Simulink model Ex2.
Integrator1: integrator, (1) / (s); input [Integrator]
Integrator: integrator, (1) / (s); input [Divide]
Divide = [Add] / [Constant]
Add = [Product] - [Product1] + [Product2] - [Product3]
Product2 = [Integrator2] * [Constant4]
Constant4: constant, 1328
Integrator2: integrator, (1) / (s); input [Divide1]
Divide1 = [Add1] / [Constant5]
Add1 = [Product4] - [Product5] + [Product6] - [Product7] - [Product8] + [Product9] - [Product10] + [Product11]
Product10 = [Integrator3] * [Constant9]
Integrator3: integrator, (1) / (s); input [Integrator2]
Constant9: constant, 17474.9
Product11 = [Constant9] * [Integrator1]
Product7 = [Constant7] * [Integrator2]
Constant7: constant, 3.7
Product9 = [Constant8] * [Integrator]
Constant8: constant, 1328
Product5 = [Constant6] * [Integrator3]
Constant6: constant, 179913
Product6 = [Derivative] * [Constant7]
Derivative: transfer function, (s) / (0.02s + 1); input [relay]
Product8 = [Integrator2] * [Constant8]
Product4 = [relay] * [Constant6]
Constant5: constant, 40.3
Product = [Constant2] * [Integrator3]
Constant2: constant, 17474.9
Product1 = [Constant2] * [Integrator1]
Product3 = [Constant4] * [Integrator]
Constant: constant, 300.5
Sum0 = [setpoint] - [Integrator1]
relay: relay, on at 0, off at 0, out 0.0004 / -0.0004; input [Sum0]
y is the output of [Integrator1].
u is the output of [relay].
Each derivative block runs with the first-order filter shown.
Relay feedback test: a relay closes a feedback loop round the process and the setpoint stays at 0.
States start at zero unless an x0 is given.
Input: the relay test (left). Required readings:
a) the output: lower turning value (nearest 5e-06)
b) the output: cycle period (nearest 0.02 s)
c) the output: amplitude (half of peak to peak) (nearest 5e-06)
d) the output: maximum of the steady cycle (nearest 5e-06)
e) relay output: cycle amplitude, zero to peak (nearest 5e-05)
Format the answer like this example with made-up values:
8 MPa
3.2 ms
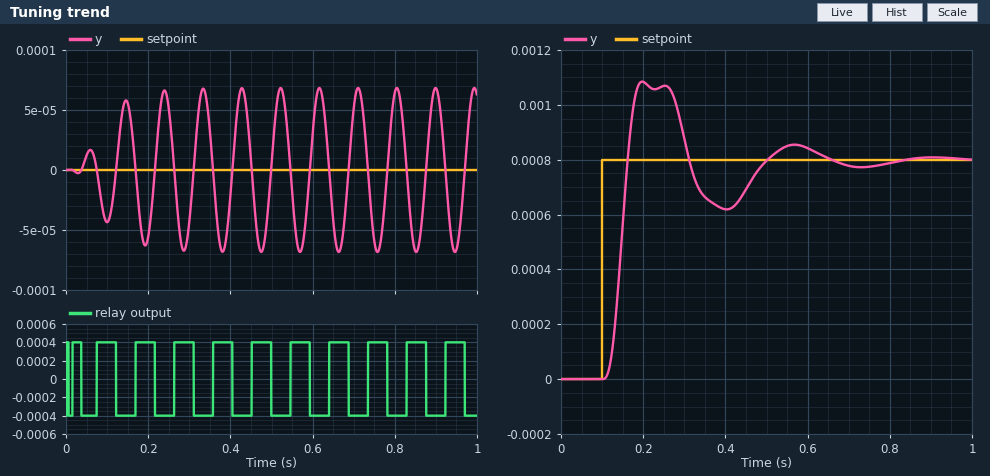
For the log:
-0.000070
0.10 s
0.000070
0.000070
0.00040
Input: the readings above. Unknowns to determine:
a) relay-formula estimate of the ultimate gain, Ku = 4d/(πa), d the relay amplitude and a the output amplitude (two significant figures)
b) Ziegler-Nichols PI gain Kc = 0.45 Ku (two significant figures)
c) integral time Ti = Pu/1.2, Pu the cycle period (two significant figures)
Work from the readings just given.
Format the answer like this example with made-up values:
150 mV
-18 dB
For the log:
7.3
3.3
0.083 s
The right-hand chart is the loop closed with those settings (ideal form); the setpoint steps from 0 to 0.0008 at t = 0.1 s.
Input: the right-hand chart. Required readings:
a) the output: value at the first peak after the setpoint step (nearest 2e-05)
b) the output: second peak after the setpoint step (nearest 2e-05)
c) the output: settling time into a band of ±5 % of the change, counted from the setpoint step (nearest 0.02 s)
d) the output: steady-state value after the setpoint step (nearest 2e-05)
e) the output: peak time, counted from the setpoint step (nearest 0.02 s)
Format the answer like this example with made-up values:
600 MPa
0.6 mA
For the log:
0.00108
0.00086
0.50 s
0.00080
0.10 s
